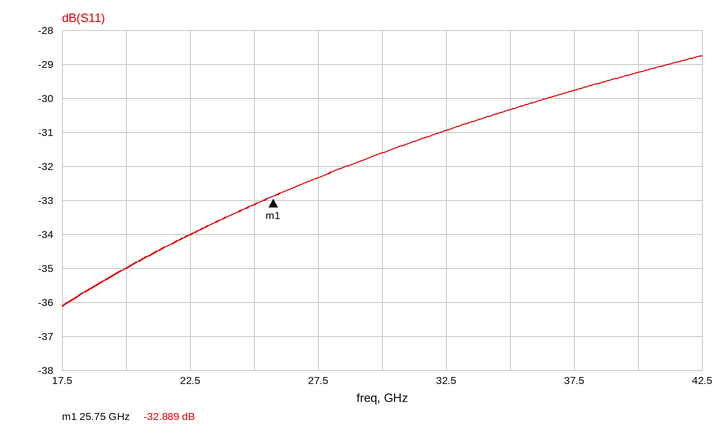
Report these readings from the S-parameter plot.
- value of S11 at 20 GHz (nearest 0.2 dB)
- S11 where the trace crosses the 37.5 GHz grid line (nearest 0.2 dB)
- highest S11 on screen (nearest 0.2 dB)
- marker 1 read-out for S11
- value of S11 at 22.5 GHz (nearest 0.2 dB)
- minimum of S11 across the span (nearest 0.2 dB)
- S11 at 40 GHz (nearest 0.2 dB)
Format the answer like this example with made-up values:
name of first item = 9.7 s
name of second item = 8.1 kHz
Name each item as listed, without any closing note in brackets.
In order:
value of S11 at 20 GHz = -35.0 dB
S11 where the trace crosses the 37.5 GHz grid line = -29.8 dB
highest S11 on screen = -28.8 dB
marker 1 read-out for S11 = -32.889 dB
value of S11 at 22.5 GHz = -34.0 dB
minimum of S11 across the span = -36.2 dB
S11 at 40 GHz = -29.2 dB
